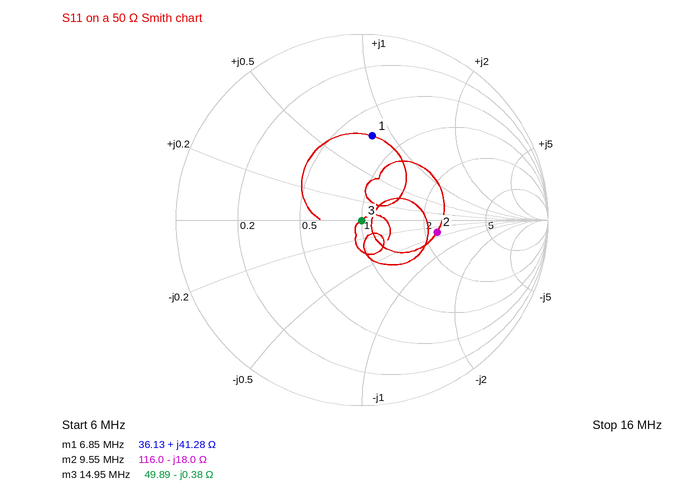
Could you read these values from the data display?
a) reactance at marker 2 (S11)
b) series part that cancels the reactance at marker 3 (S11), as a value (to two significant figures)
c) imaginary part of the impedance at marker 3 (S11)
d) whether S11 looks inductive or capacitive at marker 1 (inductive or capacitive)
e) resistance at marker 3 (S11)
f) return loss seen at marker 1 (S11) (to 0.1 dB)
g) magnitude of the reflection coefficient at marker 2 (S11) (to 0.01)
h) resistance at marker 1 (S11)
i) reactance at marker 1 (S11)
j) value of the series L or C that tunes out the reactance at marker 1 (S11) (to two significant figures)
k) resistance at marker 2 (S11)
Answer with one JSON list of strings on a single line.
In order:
["-18.0 Ω", "4.0 nH", "-0.38 Ω", "inductive", "49.89 Ω", "6.8 dB", "0.41", "36.13 Ω", "+41.28 Ω", "560 pF", "116.0 Ω"]
